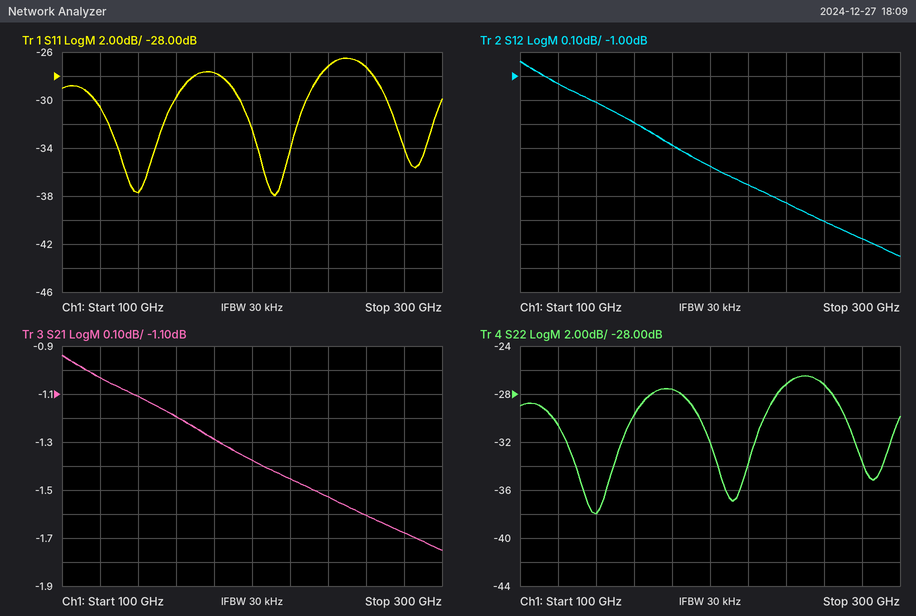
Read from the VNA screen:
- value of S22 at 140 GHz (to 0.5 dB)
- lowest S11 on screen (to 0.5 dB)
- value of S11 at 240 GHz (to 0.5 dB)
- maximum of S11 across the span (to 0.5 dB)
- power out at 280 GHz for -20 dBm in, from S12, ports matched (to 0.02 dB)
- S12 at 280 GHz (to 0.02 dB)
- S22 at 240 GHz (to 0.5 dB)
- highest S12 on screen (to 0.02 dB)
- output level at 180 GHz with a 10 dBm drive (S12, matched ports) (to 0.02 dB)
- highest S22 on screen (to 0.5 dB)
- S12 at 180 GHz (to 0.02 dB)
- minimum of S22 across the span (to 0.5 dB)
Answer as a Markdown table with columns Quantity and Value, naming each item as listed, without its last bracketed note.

| Quantity | Value |
|---|---|
| value of S22 at 140 GHz | -38.0 dB |
| lowest S11 on screen | -38.0 dB |
| value of S11 at 240 GHz | -27.0 dB |
| maximum of S11 across the span | -26.5 dB |
| power out at 280 GHz for -20 dBm in, from S12, ports matched | -21.68 dBm |
| S12 at 280 GHz | -1.68 dB |
| S22 at 240 GHz | -27.0 dB |
| highest S12 on screen | -0.94 dB |
| output level at 180 GHz with a 10 dBm drive (S12, matched ports) | 8.72 dBm |
| highest S22 on screen | -26.5 dB |
| S12 at 180 GHz | -1.28 dB |
| minimum of S22 across the span | -38.0 dB |
